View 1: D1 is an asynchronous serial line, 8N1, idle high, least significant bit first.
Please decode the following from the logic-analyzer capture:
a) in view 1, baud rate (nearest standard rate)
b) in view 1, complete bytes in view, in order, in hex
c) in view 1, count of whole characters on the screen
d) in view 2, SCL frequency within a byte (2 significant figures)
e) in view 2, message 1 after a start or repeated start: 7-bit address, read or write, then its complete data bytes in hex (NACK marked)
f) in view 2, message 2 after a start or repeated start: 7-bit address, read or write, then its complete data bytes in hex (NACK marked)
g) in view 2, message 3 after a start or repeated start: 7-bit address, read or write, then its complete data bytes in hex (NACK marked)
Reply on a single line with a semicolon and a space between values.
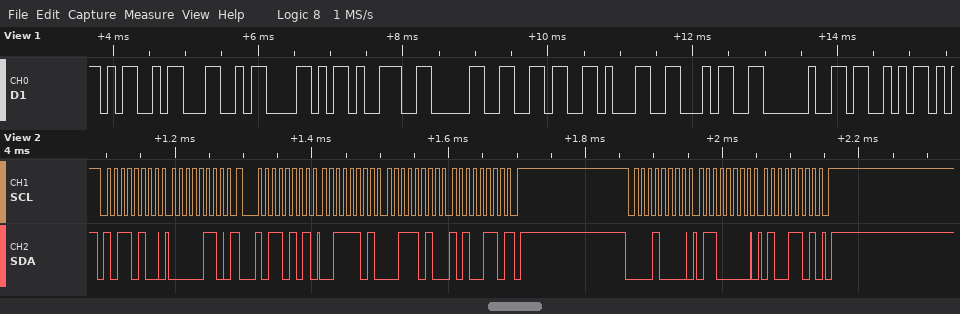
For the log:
9600 baud; 0x4D 0x4C 0x58 0x39 0x30 0x36 0x31 0x34 0x20 0x53; 10; 100 kHz; 0x5A write: 06; 0x5A read: 3D 3A A6 NACK; 0x08 write: 60 4D
